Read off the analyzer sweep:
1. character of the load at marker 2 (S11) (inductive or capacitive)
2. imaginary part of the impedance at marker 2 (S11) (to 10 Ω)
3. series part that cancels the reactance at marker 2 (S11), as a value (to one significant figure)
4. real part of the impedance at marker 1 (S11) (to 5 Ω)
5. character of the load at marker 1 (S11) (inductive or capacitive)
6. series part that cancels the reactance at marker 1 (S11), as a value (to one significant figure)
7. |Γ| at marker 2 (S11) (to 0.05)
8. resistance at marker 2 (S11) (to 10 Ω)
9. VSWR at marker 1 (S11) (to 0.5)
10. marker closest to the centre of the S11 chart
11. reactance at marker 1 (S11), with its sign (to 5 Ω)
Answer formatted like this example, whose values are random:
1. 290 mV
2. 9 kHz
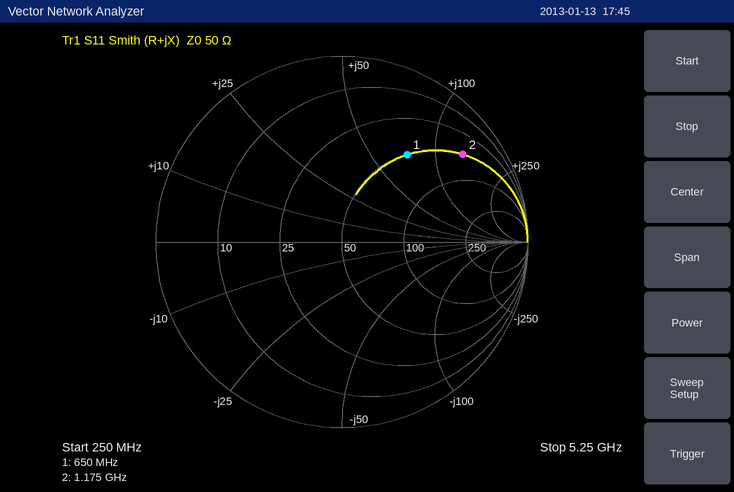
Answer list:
1. inductive
2. +140 Ω
3. 1.0 pF
4. 50 Ω
5. inductive
6. 3 pF
7. 0.80
8. 50 Ω
9. 4.0
10. marker 1
11. +75 Ω
